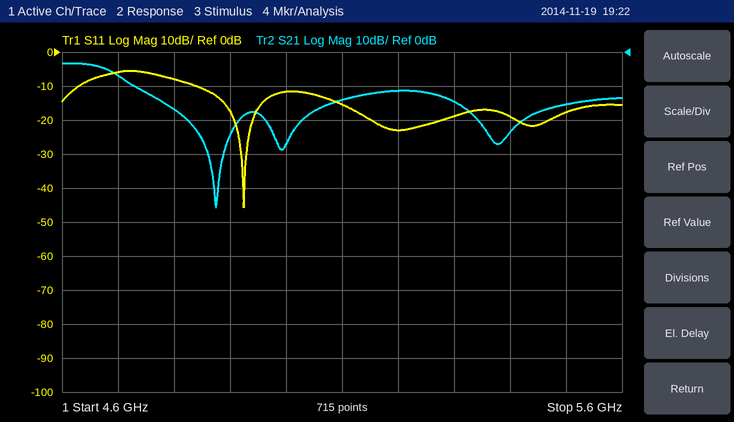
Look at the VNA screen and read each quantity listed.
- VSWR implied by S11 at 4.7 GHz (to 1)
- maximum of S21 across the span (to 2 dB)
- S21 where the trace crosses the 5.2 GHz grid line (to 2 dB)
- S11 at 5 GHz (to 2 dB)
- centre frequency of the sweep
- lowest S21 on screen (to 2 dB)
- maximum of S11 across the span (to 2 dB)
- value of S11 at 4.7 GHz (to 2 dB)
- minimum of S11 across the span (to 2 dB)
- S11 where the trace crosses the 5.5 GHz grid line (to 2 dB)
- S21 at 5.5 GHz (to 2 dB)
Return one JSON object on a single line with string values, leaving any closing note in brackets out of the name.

{"VSWR implied by S11 at 4.7 GHz": "3", "maximum of S21 across the span": "-4 dB", "S21 where the trace crosses the 5.2 GHz grid line": "-12 dB", "S11 at 5 GHz": "-12 dB", "centre frequency of the sweep": "5.1 GHz", "lowest S21 on screen": "-46 dB", "maximum of S11 across the span": "-6 dB", "value of S11 at 4.7 GHz": "-6 dB", "minimum of S11 across the span": "-46 dB", "S11 where the trace crosses the 5.5 GHz grid line": "-18 dB", "S21 at 5.5 GHz": "-16 dB"}
